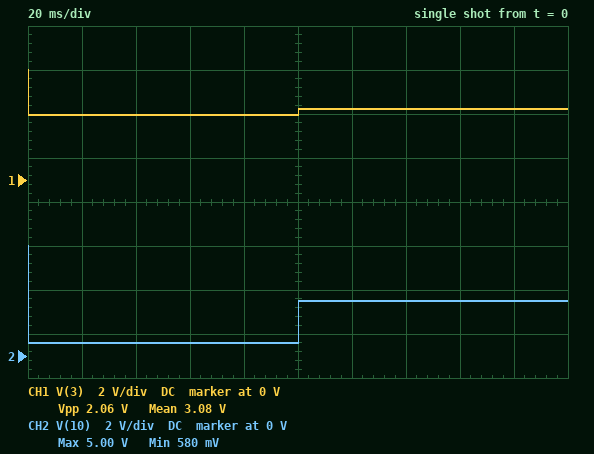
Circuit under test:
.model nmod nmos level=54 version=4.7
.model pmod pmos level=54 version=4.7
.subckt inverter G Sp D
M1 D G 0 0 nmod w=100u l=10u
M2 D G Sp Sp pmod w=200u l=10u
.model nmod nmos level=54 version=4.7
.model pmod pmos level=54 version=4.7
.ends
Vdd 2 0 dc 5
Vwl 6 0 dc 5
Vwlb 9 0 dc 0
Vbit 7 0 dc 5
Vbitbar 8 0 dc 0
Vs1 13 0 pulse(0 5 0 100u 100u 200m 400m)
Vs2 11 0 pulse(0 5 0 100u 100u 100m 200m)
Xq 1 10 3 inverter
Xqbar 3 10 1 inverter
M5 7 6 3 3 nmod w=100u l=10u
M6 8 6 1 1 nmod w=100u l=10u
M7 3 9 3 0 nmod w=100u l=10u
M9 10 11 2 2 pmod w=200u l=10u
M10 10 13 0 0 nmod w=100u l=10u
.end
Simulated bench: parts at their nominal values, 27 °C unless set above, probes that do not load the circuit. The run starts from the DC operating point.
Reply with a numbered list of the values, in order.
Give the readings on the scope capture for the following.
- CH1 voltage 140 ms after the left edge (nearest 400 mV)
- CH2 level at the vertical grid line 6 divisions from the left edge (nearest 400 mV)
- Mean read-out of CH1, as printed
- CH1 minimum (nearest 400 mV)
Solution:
1. 3.2 V
2. 2.4 V
3. 3.08 V
4. 2.8 V
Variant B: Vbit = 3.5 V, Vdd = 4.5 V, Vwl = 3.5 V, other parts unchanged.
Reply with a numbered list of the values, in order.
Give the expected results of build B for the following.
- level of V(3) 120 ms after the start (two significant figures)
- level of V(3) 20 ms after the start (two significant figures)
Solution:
1. 2.3 V
2. 2.0 V
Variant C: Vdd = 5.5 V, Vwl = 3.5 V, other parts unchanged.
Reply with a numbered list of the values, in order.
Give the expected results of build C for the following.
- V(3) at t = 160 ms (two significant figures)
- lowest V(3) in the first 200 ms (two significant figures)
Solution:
1. 2.6 V
2. 2.0 V
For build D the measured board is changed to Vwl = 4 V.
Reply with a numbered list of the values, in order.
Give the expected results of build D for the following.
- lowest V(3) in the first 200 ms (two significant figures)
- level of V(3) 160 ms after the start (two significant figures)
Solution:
1. 2.3 V
2. 2.7 V
